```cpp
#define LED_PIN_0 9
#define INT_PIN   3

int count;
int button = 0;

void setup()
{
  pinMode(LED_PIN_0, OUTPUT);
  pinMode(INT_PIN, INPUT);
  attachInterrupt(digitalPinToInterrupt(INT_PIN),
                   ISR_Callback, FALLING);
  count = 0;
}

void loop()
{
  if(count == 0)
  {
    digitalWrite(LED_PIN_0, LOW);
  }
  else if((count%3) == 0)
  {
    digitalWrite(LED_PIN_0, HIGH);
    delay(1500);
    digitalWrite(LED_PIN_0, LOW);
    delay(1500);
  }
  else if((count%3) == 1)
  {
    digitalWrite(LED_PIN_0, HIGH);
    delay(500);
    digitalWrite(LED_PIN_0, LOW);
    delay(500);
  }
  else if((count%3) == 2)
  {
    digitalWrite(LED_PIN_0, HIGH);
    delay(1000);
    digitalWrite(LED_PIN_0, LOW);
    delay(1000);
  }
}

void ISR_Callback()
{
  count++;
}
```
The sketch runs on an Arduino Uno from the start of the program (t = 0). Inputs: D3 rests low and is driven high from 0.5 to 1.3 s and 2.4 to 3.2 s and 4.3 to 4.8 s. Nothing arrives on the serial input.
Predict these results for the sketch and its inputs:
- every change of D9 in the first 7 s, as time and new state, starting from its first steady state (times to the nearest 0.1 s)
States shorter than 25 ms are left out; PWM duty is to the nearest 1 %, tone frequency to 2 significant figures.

0 s low; 1.3 s high; 1.8 s low; 2.3 s high; 2.8 s low; 3.3 s high; 4.3 s low; 5.3 s high; 6.8 s low
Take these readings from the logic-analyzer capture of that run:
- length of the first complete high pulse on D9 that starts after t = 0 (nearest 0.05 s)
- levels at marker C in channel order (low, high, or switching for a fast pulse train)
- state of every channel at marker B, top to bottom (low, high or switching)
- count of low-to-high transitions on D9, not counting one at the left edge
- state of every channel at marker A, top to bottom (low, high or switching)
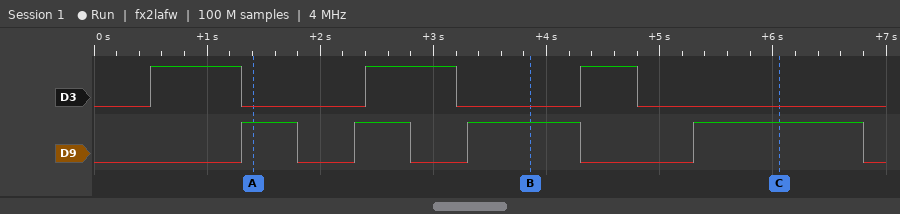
0.50 s
D3 low, D9 high
D3 low, D9 high
4
D3 low, D9 high
